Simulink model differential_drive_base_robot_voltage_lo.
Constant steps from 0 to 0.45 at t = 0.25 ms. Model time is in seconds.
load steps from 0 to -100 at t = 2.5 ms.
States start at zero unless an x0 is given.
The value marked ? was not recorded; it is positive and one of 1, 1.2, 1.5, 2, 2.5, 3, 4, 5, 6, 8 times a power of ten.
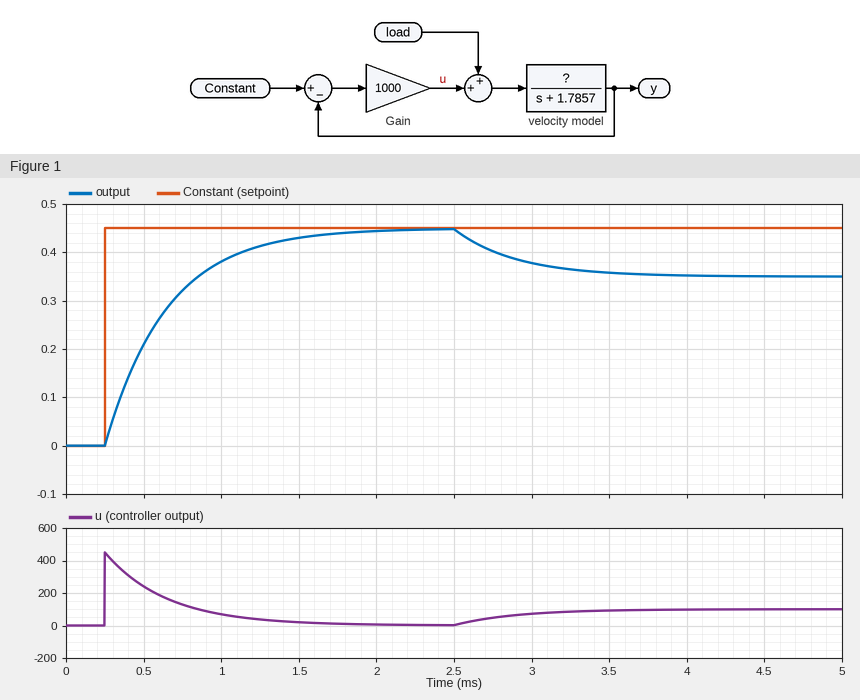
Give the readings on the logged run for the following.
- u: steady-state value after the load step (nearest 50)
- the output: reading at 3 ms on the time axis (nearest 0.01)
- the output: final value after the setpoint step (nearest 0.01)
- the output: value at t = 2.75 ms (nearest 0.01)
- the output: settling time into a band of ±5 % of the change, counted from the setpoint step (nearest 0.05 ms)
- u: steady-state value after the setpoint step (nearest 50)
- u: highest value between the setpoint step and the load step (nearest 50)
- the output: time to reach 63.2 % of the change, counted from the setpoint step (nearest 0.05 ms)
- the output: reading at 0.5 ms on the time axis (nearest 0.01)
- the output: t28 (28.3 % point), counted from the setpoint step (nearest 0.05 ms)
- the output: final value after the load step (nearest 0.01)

100
0.38
0.45
0.40
1.20 ms
0
450
0.40 ms
0.21
0.15 ms
0.35
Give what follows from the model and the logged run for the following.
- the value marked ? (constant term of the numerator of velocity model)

2.5
